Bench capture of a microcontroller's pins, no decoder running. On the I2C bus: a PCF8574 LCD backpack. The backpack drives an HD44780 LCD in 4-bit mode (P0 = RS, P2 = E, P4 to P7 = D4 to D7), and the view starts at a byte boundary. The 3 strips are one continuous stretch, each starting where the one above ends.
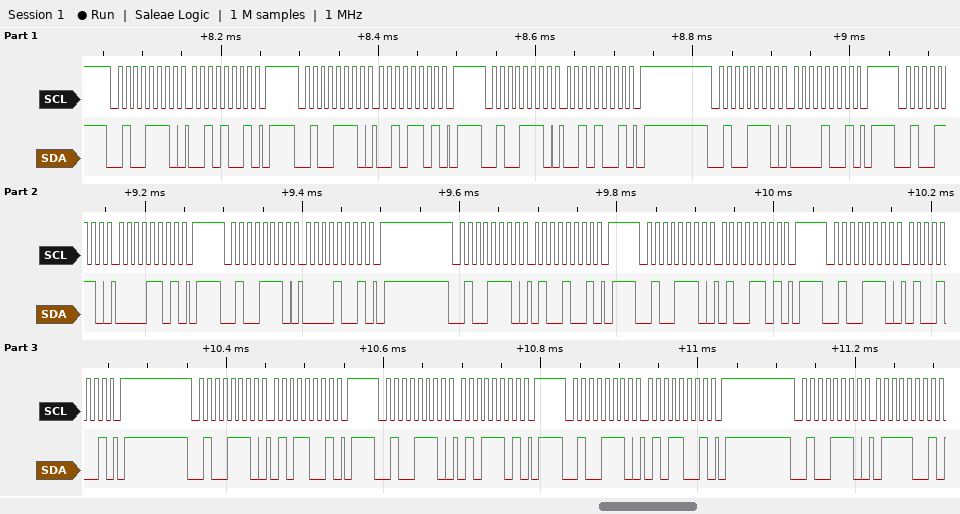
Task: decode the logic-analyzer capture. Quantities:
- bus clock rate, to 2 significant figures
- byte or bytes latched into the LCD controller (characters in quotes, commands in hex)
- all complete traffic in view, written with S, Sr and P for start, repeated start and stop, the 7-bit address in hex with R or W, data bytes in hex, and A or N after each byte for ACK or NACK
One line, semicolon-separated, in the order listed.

100 kHz; ' ' 'E'; S 27W A 29 A P S 27W A 2D A P S 27W A 29 A P S 27W A 09 A P S 27W A 0D A P S 27W A 09 A P S 27W A 49 A P S 27W A 4D A P S 27W A 49 A P S 27W A 59 A P S 27W A 5D A P S 27W A 59 A P S 27W A 79 A
